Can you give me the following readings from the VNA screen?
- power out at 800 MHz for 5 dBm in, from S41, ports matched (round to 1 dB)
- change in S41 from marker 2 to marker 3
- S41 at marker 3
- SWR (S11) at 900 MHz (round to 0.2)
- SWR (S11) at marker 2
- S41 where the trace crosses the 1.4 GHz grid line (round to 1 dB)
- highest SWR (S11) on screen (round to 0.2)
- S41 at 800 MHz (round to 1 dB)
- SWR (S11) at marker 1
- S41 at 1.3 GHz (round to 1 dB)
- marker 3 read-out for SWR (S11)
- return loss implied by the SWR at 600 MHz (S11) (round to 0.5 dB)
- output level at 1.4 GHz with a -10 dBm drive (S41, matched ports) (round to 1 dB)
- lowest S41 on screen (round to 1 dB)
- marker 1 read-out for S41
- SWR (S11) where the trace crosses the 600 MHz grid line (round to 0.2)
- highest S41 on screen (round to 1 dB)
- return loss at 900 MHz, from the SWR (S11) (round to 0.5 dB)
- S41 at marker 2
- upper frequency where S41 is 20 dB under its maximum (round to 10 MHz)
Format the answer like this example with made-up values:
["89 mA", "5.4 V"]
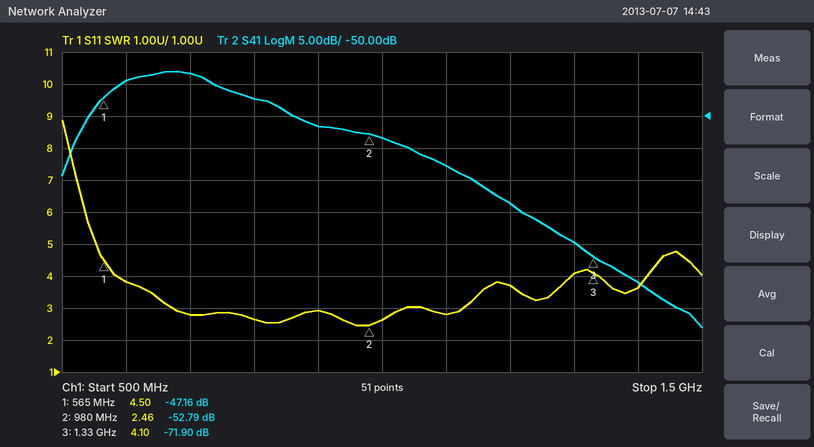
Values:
["-42 dBm", "-19.11 dB", "-71.90 dB", "3.0", "2.46", "-76 dB", "8.8", "-47 dB", "4.50", "-70 dB", "4.10", "4.5 dB", "-86 dBm", "-83 dB", "-47.16 dB", "3.8", "-43 dB", "6.0 dB", "-52.79 dB", "1.19 GHz"]
